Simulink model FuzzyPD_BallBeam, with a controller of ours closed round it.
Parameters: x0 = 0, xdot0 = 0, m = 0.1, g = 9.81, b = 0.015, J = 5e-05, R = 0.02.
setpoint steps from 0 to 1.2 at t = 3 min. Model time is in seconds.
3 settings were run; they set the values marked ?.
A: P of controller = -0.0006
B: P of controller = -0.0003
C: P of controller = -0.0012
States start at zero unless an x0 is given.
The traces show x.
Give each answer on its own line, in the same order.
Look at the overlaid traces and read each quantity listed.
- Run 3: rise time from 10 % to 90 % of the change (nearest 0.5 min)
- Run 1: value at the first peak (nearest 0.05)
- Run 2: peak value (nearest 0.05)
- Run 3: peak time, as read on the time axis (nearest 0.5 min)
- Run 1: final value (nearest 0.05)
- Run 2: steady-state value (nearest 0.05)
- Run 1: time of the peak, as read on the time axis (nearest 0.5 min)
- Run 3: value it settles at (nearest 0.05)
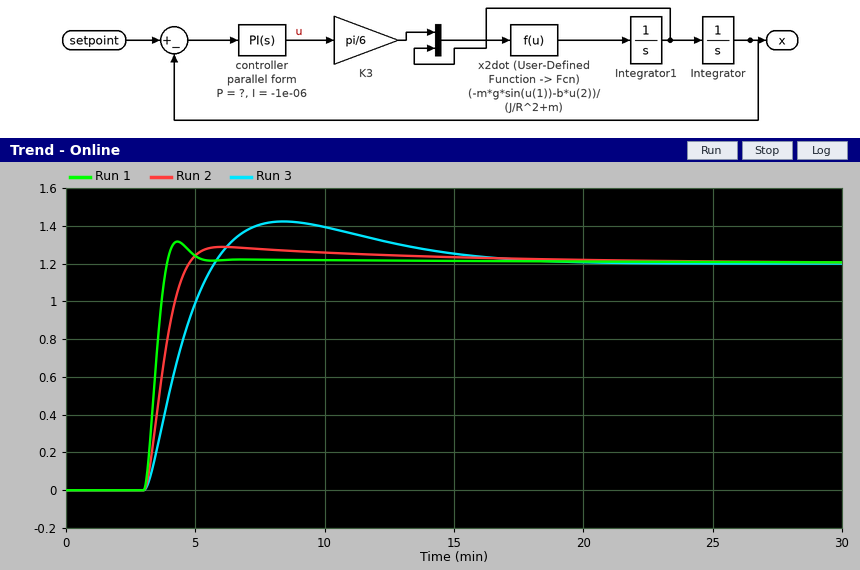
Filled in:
2.0 min
1.30
1.30
8.5 min
1.20
1.20
4.5 min
1.20
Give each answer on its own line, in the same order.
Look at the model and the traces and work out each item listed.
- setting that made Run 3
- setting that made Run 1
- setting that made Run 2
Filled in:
B
C
A
